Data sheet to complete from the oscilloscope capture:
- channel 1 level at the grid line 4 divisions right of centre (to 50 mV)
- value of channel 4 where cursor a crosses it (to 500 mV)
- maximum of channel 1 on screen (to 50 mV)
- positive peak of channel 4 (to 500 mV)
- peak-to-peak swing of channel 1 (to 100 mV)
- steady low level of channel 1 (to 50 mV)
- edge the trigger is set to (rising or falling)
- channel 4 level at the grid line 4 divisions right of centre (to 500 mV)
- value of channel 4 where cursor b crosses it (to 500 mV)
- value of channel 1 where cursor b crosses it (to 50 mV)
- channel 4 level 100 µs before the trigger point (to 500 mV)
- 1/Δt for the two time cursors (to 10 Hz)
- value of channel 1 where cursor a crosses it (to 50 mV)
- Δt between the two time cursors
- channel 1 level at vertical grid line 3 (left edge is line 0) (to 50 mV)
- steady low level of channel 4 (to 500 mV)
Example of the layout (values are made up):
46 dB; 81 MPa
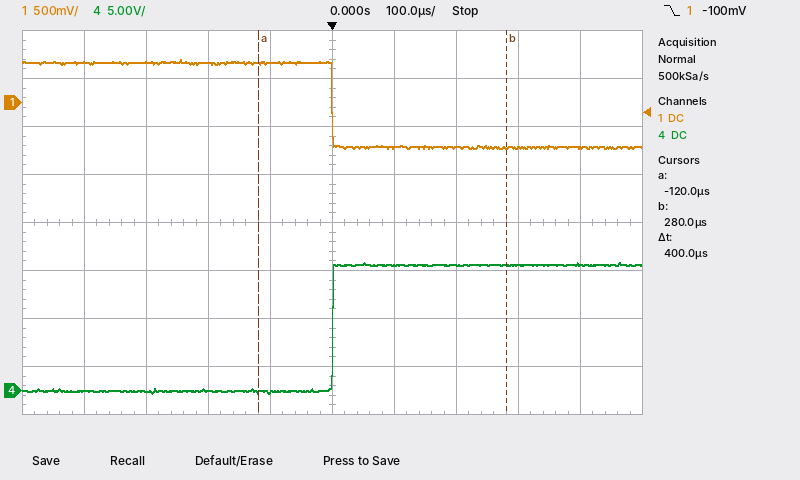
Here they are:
-450 mV; 0.0 V; 450 mV; 13.5 V; 900 mV; -450 mV; falling; 13.0 V; 13.0 V; -450 mV; 0.0 V; 2.50 kHz; 400 mV; 400 µs; 400 mV; 0.0 V
